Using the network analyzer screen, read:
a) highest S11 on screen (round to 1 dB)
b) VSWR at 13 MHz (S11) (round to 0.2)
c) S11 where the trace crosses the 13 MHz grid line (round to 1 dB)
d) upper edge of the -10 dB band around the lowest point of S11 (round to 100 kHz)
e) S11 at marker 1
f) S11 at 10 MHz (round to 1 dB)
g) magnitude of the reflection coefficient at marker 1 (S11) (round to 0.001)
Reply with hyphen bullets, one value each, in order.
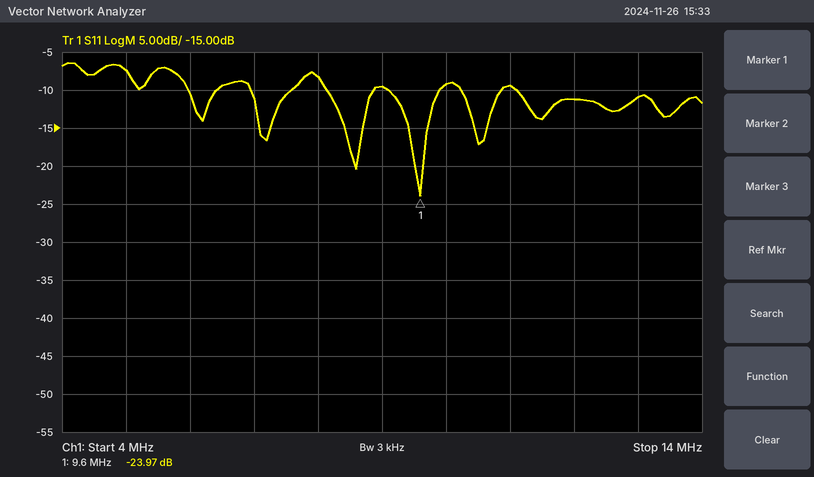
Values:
- -6 dB
- 1.8
- -11 dB
- 9.9 MHz
- -23.97 dB
- -9 dB
- 0.063
